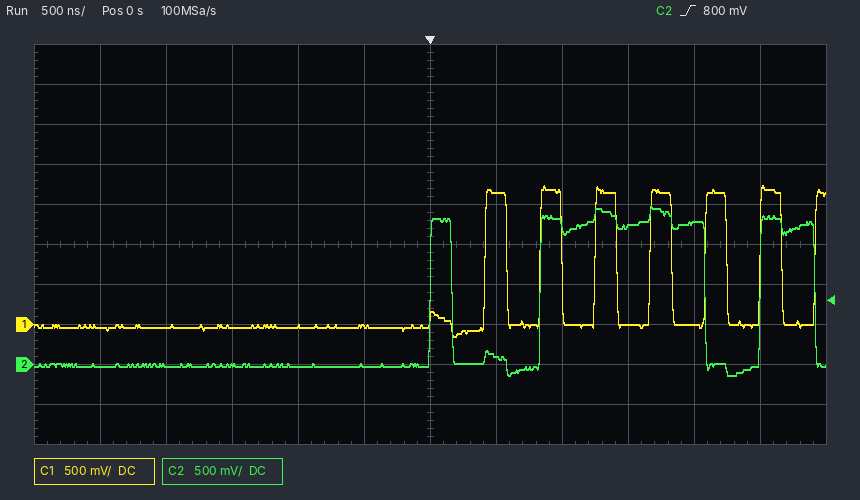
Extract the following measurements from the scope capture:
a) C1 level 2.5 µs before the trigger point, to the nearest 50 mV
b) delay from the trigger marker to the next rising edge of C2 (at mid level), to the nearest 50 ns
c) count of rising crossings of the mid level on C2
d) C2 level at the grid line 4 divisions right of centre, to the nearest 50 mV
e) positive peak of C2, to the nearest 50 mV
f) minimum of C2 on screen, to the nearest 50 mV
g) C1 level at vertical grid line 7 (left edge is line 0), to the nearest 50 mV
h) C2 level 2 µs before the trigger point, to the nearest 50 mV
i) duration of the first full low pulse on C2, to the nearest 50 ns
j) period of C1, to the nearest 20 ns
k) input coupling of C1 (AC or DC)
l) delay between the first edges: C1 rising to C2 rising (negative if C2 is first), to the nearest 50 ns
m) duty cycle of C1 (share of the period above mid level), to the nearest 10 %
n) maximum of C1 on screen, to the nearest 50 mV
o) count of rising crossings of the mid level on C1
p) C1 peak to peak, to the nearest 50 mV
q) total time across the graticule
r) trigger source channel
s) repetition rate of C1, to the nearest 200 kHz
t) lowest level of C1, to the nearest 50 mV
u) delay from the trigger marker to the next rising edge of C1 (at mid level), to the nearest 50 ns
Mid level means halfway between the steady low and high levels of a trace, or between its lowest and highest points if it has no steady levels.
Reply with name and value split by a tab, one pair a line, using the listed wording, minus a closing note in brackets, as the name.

C1 level 2.5 µs before the trigger point, to the nearest 50 mV	-50 mV
delay from the trigger marker to the next rising edge of C2 (at mid level), to the nearest 50 ns	850 ns
count of rising crossings of the mid level on C2	3
C2 level at the grid line 4 divisions right of centre, to the nearest 50 mV	1.75 V
positive peak of C2, to the nearest 50 mV	2.00 V
minimum of C2 on screen, to the nearest 50 mV	-150 mV
C1 level at vertical grid line 7 (left edge is line 0), to the nearest 50 mV	1.65 V
C2 level 2 µs before the trigger point, to the nearest 50 mV	0 mV
duration of the first full low pulse on C2, to the nearest 50 ns	650 ns
period of C1, to the nearest 20 ns	420 ns
input coupling of C1	DC
delay between the first edges: C1 rising to C2 rising (negative if C2 is first), to the nearest 50 ns	-400 ns
duty cycle of C1 (share of the period above mid level), to the nearest 10 %	40 %
maximum of C1 on screen, to the nearest 50 mV	1.75 V
count of rising crossings of the mid level on C1	7
C1 peak to peak, to the nearest 50 mV	1.90 V
total time across the graticule	6 µs
trigger source channel	C2
repetition rate of C1, to the nearest 200 kHz	2.4 MHz
lowest level of C1, to the nearest 50 mV	-150 mV
delay from the trigger marker to the next rising edge of C1 (at mid level), to the nearest 50 ns	400 ns
